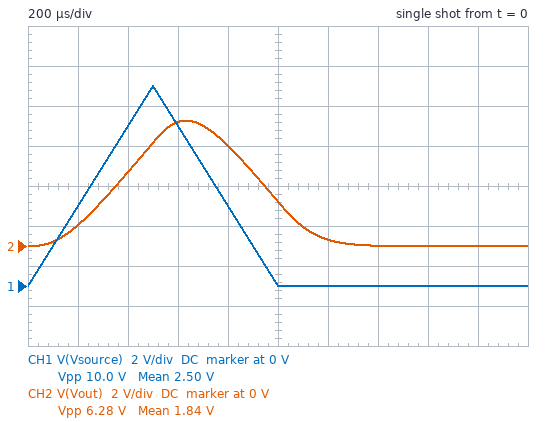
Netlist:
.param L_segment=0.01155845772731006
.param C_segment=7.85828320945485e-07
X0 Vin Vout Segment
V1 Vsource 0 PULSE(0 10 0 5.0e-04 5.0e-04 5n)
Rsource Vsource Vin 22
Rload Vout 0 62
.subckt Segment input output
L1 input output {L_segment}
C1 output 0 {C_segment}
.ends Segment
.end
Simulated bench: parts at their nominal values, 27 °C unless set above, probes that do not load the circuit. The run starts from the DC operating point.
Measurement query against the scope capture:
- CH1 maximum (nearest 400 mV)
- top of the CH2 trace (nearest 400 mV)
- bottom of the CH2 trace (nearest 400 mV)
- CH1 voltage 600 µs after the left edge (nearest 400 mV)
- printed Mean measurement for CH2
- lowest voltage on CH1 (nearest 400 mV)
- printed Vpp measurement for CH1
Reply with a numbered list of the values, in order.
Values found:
1. 10.0 V
2. 6.4 V
3. 0 V
4. 8.0 V
5. 1.84 V
6. 0 V
7. 10.0 V
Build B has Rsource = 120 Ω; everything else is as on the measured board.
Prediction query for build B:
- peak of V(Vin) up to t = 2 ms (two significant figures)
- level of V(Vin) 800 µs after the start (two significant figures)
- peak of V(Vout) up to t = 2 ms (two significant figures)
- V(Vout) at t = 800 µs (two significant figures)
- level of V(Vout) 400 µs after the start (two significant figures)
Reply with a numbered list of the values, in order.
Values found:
1. 4.0 V
2. 730 mV
3. 3.1 V
4. 2.0 V
5. 2.1 V
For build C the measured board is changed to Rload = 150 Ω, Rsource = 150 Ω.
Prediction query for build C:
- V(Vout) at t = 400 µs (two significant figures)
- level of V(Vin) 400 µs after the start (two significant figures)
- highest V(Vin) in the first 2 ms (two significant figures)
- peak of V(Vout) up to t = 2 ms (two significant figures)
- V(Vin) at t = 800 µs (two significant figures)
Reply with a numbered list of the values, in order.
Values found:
1. 3.0 V
2. 3.8 V
3. 4.8 V
4. 4.6 V
5. 2.2 V
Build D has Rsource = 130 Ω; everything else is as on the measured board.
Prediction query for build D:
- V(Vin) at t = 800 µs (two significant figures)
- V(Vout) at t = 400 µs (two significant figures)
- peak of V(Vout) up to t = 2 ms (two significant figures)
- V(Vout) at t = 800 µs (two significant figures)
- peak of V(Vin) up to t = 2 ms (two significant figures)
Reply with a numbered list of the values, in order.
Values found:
1. 680 mV
2. 2.0 V
3. 2.9 V
4. 1.9 V
5. 3.8 V
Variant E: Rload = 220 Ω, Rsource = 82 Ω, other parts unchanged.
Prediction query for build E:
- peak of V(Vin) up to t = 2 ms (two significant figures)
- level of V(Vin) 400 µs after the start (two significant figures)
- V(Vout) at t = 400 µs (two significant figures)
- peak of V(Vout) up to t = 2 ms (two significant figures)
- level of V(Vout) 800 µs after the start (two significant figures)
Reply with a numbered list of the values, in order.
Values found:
1. 6.8 V
2. 5.3 V
3. 4.6 V
4. 7.0 V
5. 4.5 V
